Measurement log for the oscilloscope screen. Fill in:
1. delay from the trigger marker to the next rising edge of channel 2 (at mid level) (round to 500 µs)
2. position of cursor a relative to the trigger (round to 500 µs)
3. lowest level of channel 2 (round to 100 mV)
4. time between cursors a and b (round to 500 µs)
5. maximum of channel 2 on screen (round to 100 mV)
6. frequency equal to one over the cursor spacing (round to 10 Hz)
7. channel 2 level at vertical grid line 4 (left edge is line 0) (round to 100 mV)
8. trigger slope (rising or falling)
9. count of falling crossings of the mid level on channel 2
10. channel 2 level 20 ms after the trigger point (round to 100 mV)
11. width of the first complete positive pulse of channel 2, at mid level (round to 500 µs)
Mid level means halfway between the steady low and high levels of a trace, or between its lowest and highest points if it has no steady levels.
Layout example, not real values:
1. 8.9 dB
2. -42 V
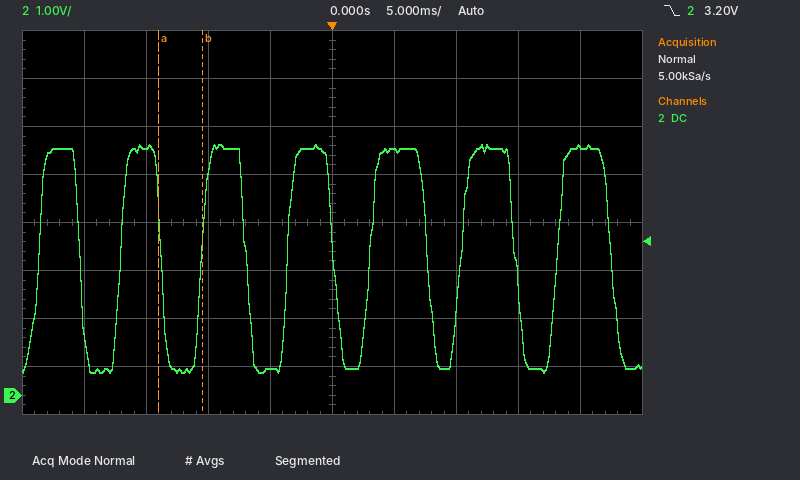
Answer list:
1. 3.0 ms
2. -14.0 ms
3. 500 mV
4. 3.5 ms
5. 5.2 V
6. 290 Hz
7. 600 mV
8. falling
9. 7
10. 5.2 V
11. 3.5 ms
